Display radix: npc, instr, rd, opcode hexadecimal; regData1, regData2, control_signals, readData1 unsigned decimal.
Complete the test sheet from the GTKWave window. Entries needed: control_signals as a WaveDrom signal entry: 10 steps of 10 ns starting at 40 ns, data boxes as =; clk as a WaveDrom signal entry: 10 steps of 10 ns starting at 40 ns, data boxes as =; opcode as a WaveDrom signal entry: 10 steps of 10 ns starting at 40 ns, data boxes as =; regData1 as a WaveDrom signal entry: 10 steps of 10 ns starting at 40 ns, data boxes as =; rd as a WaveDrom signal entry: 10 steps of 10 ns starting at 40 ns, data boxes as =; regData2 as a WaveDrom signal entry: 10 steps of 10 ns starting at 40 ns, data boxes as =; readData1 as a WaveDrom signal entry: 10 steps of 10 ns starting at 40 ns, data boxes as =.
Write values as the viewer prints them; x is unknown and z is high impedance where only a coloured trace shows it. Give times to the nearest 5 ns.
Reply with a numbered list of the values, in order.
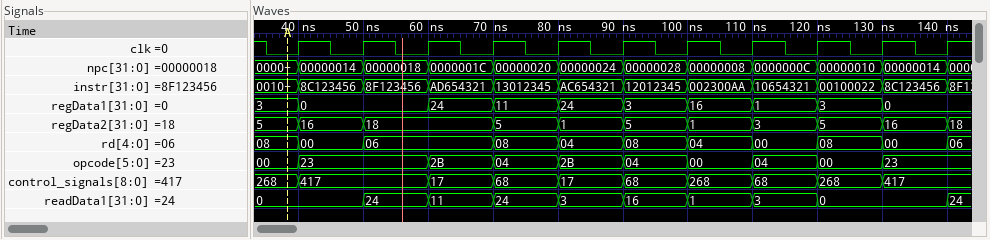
1. {name: 'control_signals', wave: '=.========', data: '417 17 68 17 68 268 68 268 417'}
2. {name: 'clk', wave: 'p.........'}
3. {name: 'opcode', wave: '=.========', data: '23 2B 04 2B 04 00 04 00 23'}
4. {name: 'regData1', wave: '=.========', data: '0 24 11 24 3 16 1 3 0'}
5. {name: 'rd', wave: '==.=======', data: '00 06 08 04 08 04 00 08 00'}
6. {name: 'regData2', wave: '==.=======', data: '16 18 5 1 5 1 3 5 16'}
7. {name: 'readData1', wave: '=========.', data: '0 24 11 24 3 16 1 3 0'}
